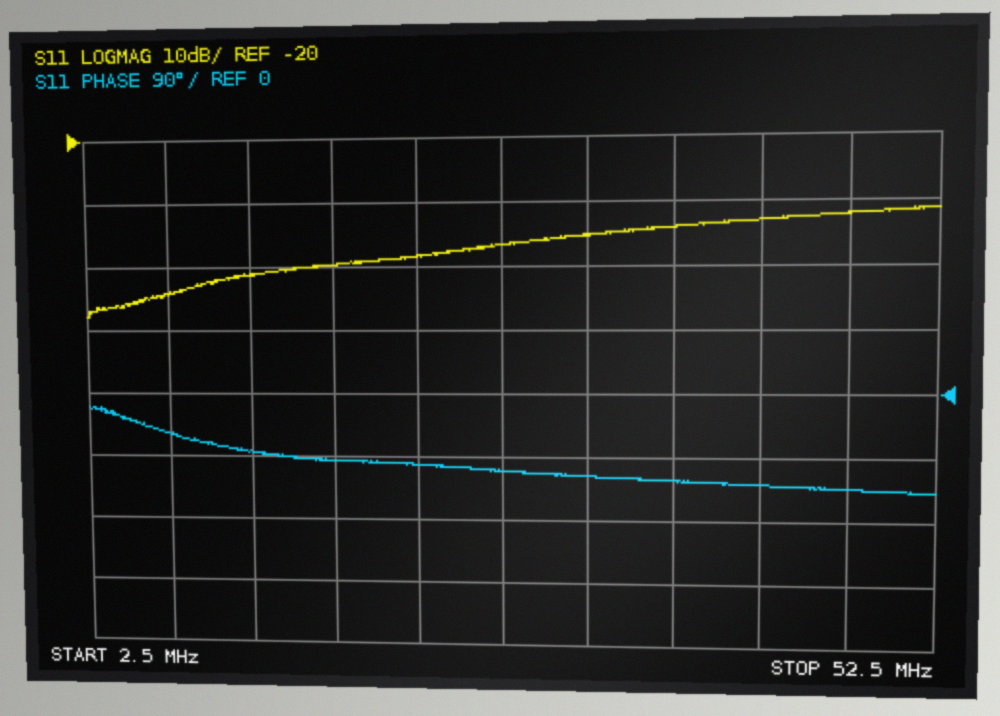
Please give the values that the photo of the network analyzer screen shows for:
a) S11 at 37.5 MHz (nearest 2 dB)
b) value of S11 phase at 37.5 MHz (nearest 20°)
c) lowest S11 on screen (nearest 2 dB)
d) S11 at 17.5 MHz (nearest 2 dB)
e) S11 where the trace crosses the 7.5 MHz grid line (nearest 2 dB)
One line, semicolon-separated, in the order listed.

-34 dB; -120°; -48 dB; -40 dB; -44 dB
